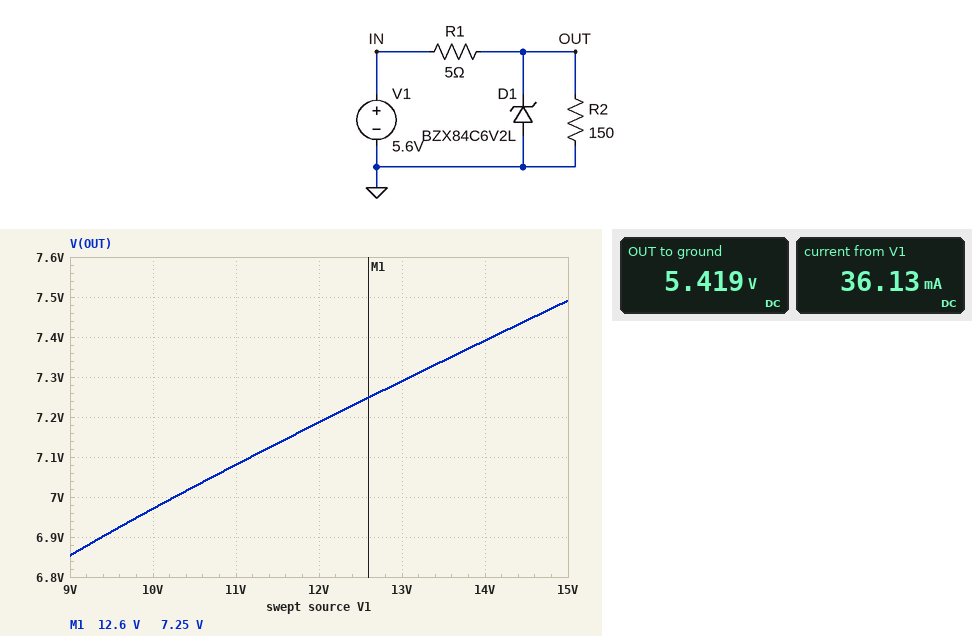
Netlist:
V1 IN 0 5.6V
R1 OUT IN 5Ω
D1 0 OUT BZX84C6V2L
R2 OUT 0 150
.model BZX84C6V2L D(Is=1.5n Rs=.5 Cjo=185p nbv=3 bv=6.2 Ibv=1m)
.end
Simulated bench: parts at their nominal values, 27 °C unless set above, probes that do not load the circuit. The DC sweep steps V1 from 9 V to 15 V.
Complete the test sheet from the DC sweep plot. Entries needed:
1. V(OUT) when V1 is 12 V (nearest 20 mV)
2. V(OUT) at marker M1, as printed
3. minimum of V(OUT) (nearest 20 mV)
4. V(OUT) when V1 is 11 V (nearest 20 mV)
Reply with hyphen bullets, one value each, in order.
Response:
- 7.18 V
- 7.25 V
- 6.86 V
- 7.08 V
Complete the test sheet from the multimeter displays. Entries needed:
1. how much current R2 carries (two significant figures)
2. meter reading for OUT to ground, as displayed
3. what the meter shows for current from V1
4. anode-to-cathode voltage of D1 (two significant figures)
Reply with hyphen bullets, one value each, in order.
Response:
- 36 mA
- 5.419 V
- 36.13 mA
- -5.4 V
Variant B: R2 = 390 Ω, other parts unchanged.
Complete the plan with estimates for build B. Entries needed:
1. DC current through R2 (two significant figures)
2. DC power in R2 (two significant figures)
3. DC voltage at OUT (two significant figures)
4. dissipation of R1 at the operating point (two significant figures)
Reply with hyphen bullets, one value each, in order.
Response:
- 14 mA
- 78 mW
- 5.5 V
- 1.0 mW
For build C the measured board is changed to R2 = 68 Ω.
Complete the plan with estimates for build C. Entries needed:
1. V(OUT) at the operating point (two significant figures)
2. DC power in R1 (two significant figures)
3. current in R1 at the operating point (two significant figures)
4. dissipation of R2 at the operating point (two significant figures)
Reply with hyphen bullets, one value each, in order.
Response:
- 5.2 V
- 29 mW
- 77 mA
- 400 mW
